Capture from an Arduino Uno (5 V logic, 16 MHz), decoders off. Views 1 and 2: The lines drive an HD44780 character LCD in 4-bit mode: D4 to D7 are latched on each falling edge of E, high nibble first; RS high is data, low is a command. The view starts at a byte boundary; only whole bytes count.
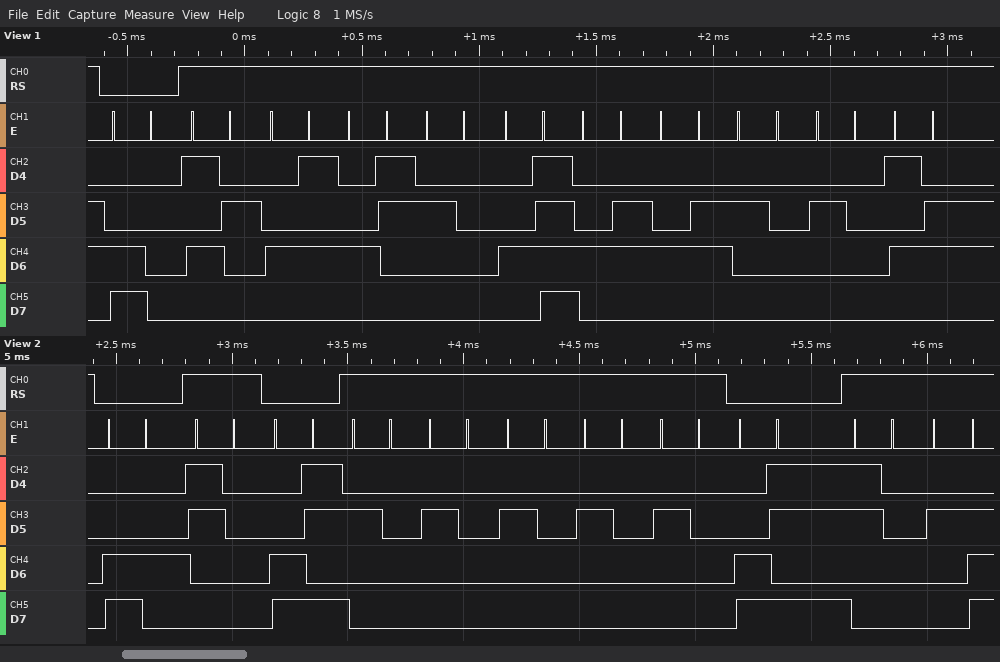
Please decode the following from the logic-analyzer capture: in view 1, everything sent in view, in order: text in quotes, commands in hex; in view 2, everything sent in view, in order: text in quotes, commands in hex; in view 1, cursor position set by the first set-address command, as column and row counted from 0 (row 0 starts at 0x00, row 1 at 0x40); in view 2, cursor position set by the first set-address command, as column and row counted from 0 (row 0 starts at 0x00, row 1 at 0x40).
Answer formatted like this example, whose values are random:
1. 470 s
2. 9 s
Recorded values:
1. 0xC0 "REC OFF  V"
2. 0xC4 "0" 0xCB "     " 0xCB "0."
3. column 0, row 1
4. column 4, row 1
